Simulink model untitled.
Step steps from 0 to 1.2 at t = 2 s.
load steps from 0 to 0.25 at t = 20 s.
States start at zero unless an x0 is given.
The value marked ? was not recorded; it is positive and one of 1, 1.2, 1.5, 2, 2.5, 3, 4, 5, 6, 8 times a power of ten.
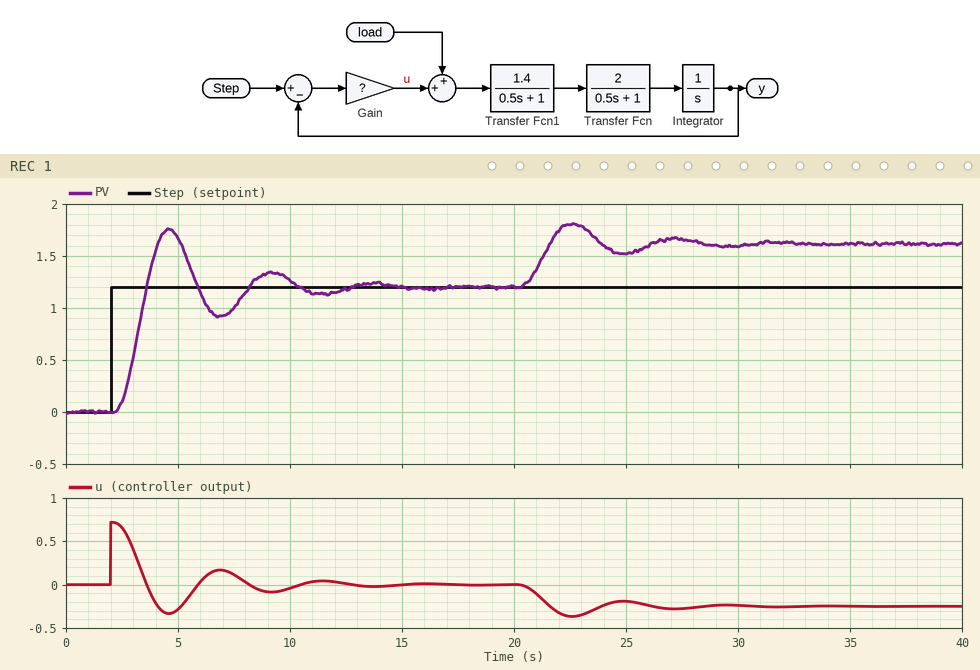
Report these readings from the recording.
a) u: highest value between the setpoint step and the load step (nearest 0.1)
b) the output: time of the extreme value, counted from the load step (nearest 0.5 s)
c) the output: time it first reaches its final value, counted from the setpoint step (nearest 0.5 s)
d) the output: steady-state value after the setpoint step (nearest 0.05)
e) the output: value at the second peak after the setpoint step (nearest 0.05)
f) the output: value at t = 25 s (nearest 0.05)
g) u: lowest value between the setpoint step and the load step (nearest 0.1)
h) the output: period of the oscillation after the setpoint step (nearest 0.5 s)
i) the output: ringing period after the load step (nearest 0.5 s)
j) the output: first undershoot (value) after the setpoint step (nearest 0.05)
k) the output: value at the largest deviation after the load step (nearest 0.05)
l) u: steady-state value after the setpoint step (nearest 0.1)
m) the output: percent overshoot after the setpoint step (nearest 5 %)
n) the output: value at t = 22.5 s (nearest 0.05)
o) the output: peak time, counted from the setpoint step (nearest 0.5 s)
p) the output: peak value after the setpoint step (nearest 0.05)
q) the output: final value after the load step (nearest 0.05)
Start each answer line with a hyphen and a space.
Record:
- 0.7
- 2.5 s
- 1.5 s
- 1.20
- 1.35
- 1.50
- -0.3
- 4.5 s
- 4.5 s
- 0.90
- 1.80
- 0.0
- 45 %
- 1.80
- 2.5 s
- 1.75
- 1.60
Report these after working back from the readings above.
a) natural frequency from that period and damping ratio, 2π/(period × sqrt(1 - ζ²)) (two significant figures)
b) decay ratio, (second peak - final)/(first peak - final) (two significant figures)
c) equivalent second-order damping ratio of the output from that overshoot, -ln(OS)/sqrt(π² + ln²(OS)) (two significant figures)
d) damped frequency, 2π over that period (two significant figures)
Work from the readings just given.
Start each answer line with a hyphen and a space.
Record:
- 1.4 rad/s
- 0.27
- 0.25
- 1.4 rad/s
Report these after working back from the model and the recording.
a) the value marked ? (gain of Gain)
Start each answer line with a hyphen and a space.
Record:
- 0.6
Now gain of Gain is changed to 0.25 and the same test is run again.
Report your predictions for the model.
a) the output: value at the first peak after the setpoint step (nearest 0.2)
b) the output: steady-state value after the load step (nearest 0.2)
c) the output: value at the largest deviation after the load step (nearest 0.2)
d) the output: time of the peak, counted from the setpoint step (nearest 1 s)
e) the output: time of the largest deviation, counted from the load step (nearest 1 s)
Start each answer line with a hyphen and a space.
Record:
- 1.4
- 2.2
- 2.4
- 4 s
- 4 s
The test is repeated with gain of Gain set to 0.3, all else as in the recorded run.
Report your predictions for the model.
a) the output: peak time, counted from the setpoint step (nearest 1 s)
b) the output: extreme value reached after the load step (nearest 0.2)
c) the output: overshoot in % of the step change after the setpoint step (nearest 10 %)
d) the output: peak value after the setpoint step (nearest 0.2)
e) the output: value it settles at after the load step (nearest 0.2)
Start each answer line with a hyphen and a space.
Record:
- 4 s
- 2.2
- 20 %
- 1.4
- 2.0
